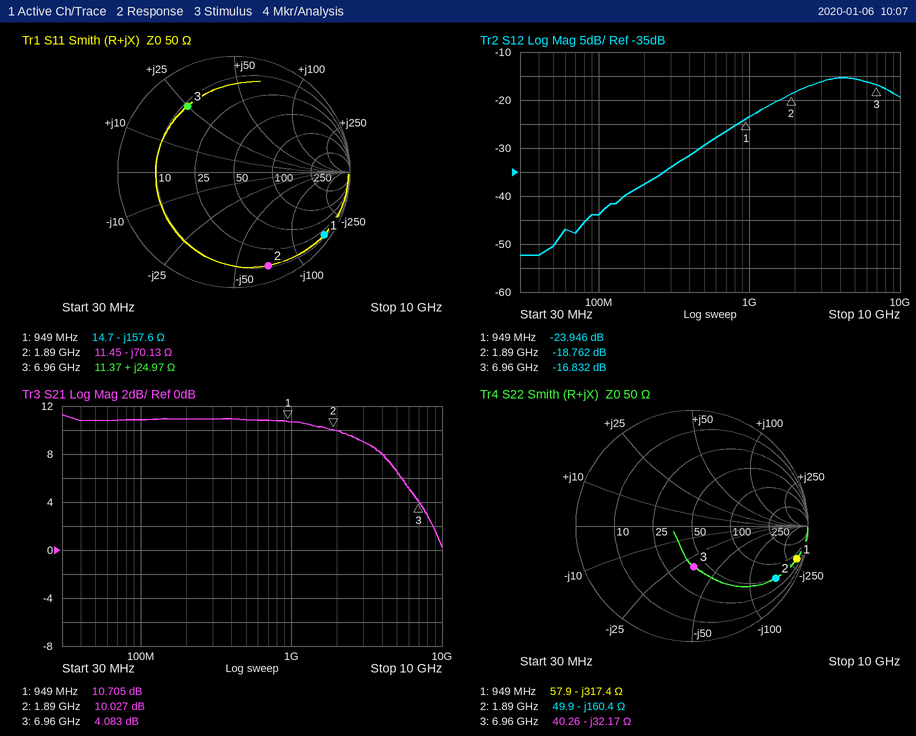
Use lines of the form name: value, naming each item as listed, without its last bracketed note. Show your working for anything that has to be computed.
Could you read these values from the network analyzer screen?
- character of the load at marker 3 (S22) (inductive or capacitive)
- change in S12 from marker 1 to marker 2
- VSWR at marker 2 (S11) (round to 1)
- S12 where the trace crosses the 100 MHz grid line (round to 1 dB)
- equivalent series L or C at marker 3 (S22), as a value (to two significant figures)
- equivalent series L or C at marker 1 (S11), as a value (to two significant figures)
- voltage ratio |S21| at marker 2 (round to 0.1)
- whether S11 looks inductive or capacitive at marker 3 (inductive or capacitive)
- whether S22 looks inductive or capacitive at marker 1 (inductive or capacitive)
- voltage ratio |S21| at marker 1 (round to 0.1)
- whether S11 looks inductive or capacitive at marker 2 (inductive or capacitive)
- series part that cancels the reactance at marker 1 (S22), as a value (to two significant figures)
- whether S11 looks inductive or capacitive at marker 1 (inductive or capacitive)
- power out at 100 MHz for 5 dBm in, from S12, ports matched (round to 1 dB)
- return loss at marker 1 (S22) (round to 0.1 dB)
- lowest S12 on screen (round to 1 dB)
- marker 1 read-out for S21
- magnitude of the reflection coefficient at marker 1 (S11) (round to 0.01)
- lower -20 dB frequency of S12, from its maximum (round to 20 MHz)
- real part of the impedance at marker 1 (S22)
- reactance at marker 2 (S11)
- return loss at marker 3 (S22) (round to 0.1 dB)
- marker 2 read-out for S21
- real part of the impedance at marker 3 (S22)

character of the load at marker 3 (S22): capacitive
change in S12 from marker 1 to marker 2: -18.762 − (-23.946) = 5.184 dB
VSWR at marker 2 (S11): 13
S12 where the trace crosses the 100 MHz grid line: -44 dB
equivalent series L or C at marker 3 (S22), as a value: C = 1/(2π × 6.96 GHz × 32.17 Ω) ≈ 711 fF, so 710 fF to two significant figures
equivalent series L or C at marker 1 (S11), as a value: C = 1/(2π × 949 MHz × 157.6 Ω) ≈ 1.1 pF
voltage ratio |S21| at marker 2: 10^(10.027/20) ≈ 3.2
whether S11 looks inductive or capacitive at marker 3: inductive
whether S22 looks inductive or capacitive at marker 1: capacitive
voltage ratio |S21| at marker 1: 10^(10.705/20) ≈ 3.4
whether S11 looks inductive or capacitive at marker 2: capacitive
series part that cancels the reactance at marker 1 (S22), as a value: L = 317.4 Ω/(2π × 949 MHz) ≈ 53 nH
whether S11 looks inductive or capacitive at marker 1: capacitive
power out at 100 MHz for 5 dBm in, from S12, ports matched: 5 dBm + (-44 dB) = -39 dBm
return loss at marker 1 (S22): 0.5 dB
lowest S12 on screen: -52 dB
marker 1 read-out for S21: 10.705 dB
magnitude of the reflection coefficient at marker 1 (S11): 0.95
lower -20 dB frequency of S12, from its maximum: 260 MHz
real part of the impedance at marker 1: 57.9 Ω
reactance at marker 2: -70.13 Ω
return loss at marker 3 (S22): 9.1 dB
marker 2 read-out for S21: 10.027 dB
real part of the impedance at marker 3: 40.26 Ω
